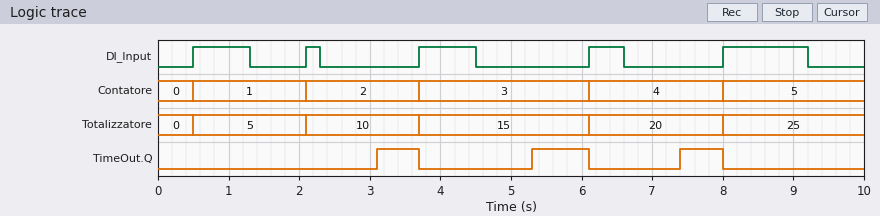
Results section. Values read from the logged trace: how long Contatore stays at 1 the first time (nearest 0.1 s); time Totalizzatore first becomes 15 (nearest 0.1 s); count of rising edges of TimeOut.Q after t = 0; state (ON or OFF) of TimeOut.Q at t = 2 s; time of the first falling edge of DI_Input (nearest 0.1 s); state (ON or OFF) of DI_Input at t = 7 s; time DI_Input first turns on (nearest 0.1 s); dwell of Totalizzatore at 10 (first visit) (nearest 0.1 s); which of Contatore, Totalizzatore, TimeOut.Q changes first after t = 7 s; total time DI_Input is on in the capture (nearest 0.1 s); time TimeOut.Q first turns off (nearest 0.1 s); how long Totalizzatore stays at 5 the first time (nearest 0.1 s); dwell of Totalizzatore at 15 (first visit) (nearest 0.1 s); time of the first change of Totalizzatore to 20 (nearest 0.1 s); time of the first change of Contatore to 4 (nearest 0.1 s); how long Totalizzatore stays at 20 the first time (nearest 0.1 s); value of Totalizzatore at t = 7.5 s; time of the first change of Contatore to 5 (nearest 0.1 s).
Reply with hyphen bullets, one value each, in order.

- 1.6 s
- 3.7 s
- 3
- OFF
- 1.3 s
- OFF
- 0.5 s
- 1.6 s
- TimeOut.Q
- 3.5 s
- 3.7 s
- 1.6 s
- 2.4 s
- 6.1 s
- 6.1 s
- 1.9 s
- 20
- 8.0 s
